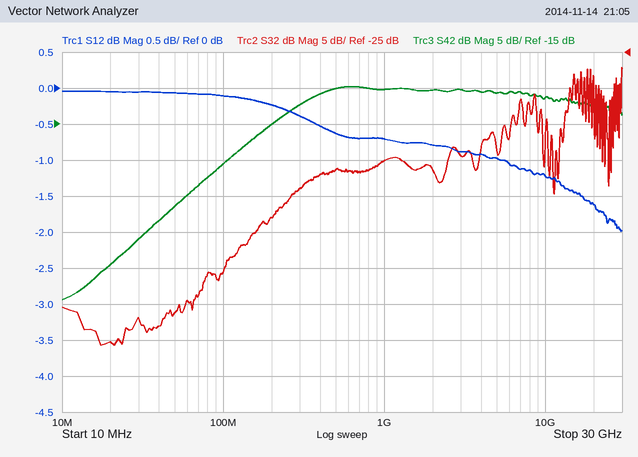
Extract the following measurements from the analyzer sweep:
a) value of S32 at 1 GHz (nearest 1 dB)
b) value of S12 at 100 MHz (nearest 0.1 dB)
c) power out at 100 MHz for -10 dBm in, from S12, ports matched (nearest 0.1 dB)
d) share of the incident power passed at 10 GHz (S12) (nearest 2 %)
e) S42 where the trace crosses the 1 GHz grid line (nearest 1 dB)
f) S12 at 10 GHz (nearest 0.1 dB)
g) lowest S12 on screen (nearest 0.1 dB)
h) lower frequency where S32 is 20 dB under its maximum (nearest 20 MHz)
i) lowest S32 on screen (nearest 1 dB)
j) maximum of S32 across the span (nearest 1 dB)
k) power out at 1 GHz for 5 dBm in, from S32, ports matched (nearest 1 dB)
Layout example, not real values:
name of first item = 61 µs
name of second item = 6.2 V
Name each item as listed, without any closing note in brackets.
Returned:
value of S32 at 1 GHz = -40 dB
value of S12 at 100 MHz = -0.1 dB
power out at 100 MHz for -10 dBm in, from S12, ports matched = -10.1 dBm
share of the incident power passed at 10 GHz (S12) = 76 %
S42 where the trace crosses the 1 GHz grid line = -10 dB
S12 at 10 GHz = -1.2 dB
lowest S12 on screen = -2.0 dB
lower frequency where S32 is 20 dB under its maximum = 220 MHz
lowest S32 on screen = -66 dB
maximum of S32 across the span = -27 dB
power out at 1 GHz for 5 dBm in, from S32, ports matched = -35 dBm
